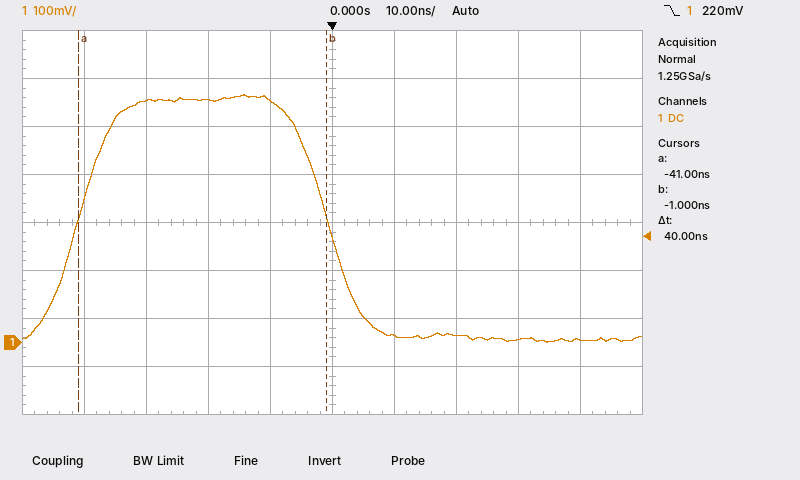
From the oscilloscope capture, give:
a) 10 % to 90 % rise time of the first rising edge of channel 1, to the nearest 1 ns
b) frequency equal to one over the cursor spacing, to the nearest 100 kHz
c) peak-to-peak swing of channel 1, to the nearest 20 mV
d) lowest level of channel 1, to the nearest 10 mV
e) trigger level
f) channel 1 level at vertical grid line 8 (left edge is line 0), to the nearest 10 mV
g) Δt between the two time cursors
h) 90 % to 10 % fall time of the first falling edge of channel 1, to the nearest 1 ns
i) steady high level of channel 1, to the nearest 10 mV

11 ns
25.0 MHz
520 mV
0 mV
220 mV
10 mV
40 ns
11 ns
510 mV
